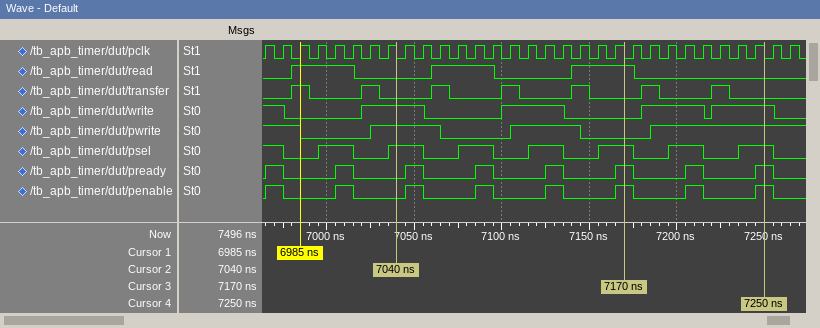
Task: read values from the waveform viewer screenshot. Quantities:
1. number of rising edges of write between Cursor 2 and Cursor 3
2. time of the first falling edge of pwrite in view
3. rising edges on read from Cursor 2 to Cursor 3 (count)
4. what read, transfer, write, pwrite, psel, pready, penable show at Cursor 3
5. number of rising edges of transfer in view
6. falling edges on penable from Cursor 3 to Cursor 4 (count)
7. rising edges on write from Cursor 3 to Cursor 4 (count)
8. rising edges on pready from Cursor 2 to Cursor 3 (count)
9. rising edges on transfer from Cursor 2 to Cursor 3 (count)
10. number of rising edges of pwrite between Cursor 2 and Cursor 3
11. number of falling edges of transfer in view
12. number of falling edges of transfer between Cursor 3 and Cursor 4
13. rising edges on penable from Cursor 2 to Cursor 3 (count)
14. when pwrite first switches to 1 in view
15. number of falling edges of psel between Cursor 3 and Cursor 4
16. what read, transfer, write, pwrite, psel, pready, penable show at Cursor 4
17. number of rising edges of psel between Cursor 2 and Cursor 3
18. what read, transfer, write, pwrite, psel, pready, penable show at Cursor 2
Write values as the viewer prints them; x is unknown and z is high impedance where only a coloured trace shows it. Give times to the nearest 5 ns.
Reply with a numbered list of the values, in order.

1. 1
2. 6985 ns
3. 2
4. read=1, transfer=0, write=0, pwrite=0, psel=1, pready=1, penable=1
5. 7
6. 2
7. 2
8. 4
9. 3
10. 1
11. 7
12. 2
13. 4
14. 7025 ns
15. 2
16. read=0, transfer=0, write=1, pwrite=1, psel=1, pready=1, penable=1
17. 3
18. read=0, transfer=0, write=1, pwrite=1, psel=1, pready=0, penable=0
